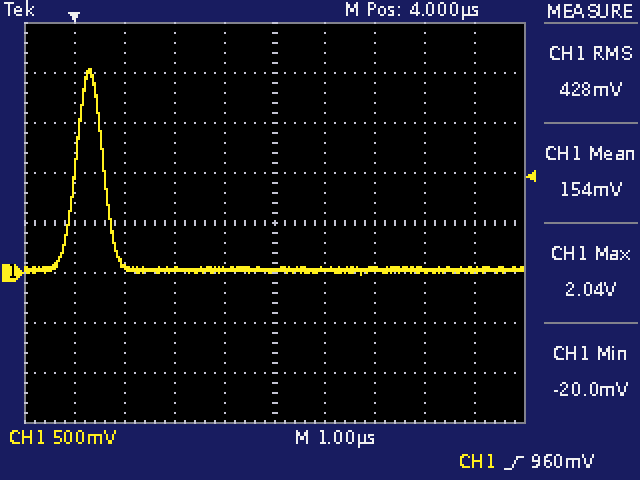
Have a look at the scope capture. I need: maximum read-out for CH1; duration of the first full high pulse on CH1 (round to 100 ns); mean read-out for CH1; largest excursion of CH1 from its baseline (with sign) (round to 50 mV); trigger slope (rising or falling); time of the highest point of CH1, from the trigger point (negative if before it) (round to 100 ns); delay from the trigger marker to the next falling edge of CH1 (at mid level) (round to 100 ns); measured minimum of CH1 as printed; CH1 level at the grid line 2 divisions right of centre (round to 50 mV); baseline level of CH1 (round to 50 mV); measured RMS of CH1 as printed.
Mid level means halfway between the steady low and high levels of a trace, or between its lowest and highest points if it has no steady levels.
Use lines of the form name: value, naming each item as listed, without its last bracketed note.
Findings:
maximum read-out for CH1: 2.04 V
duration of the first full high pulse on CH1: 600 ns
mean read-out for CH1: 154 mV
largest excursion of CH1 from its baseline (with sign): +2.00 V
trigger slope: rising
time of the highest point of CH1, from the trigger point (negative if before it): +300 ns
delay from the trigger marker to the next falling edge of CH1 (at mid level): 600 ns
measured minimum of CH1 as printed: -20.0 mV
CH1 level at the grid line 2 divisions right of centre: 50 mV
baseline level of CH1: 50 mV
measured RMS of CH1 as printed: 428 mV
